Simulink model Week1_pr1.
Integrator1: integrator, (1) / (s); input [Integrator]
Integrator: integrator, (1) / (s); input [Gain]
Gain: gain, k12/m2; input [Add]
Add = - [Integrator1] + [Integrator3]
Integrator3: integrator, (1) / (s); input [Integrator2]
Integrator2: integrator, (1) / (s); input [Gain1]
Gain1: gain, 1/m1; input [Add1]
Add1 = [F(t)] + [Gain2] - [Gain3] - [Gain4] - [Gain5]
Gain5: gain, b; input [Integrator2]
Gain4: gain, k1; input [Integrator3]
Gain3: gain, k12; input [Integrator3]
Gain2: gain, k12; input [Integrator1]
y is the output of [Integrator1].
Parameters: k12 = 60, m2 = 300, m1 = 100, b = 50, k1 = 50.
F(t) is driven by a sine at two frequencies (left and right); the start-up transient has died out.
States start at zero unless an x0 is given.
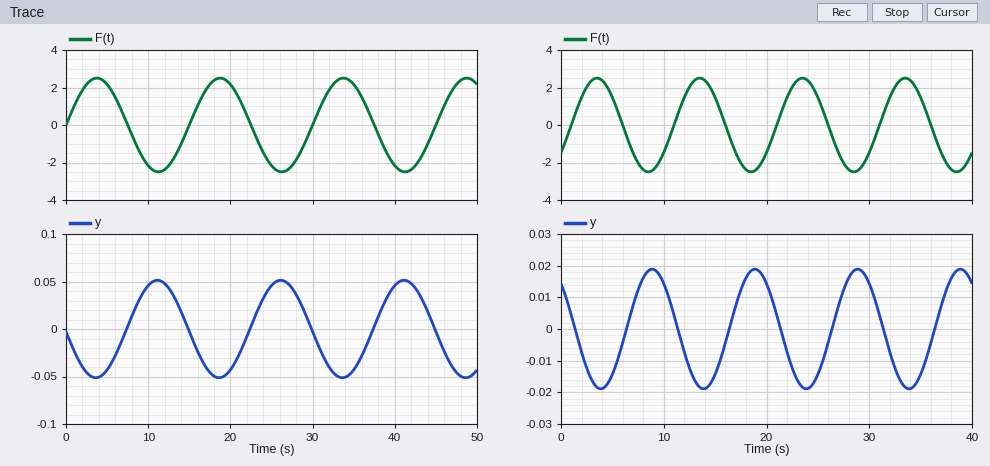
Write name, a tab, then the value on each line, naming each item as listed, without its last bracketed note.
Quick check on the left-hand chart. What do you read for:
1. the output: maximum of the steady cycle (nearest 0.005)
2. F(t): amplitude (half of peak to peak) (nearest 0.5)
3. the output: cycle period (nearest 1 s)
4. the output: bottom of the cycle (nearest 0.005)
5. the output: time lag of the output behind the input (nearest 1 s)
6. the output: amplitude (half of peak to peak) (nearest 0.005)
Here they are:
the output: maximum of the steady cycle	0.050
F(t): amplitude (half of peak to peak)	2.5
the output: cycle period	15 s
the output: bottom of the cycle	-0.050
the output: time lag of the output behind the input	7 s
the output: amplitude (half of peak to peak)	0.050
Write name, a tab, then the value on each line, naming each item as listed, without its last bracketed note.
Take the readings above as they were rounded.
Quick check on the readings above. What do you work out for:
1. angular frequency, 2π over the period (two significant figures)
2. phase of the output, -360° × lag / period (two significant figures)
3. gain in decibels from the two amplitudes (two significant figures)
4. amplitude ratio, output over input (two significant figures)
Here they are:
angular frequency, 2π over the period	0.42 rad/s
phase of the output, -360° × lag / period	-170°
gain in decibels from the two amplitudes	-34 dB
amplitude ratio, output over input	0.020
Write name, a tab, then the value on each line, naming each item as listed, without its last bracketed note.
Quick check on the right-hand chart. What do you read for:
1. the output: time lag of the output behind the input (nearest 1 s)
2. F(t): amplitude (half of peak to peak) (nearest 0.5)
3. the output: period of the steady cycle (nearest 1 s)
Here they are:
the output: time lag of the output behind the input	5 s
F(t): amplitude (half of peak to peak)	2.5
the output: period of the steady cycle	10 s
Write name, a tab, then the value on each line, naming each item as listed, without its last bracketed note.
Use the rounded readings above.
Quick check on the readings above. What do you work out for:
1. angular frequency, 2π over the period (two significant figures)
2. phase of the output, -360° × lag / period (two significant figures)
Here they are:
angular frequency, 2π over the period	0.63 rad/s
phase of the output, -360° × lag / period	-180°
